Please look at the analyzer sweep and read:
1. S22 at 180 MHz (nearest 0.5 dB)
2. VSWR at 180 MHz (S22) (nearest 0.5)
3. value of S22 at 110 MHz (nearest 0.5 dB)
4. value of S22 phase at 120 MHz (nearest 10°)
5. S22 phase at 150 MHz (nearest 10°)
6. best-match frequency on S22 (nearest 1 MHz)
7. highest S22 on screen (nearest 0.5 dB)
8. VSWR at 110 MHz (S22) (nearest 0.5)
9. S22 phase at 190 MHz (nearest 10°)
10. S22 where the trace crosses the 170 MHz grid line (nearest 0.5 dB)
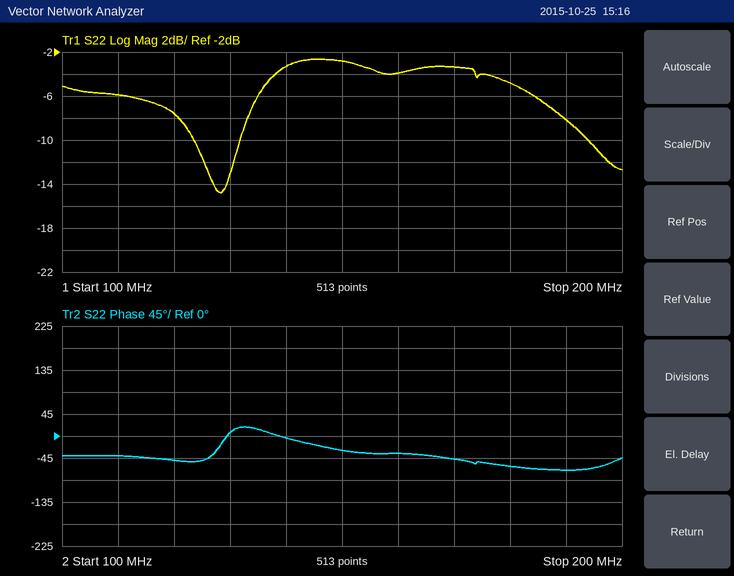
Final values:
-5.0 dB
3.5
-6.0 dB
-50°
-30°
128 MHz
-2.5 dB
3.0
-70°
-3.5 dB
